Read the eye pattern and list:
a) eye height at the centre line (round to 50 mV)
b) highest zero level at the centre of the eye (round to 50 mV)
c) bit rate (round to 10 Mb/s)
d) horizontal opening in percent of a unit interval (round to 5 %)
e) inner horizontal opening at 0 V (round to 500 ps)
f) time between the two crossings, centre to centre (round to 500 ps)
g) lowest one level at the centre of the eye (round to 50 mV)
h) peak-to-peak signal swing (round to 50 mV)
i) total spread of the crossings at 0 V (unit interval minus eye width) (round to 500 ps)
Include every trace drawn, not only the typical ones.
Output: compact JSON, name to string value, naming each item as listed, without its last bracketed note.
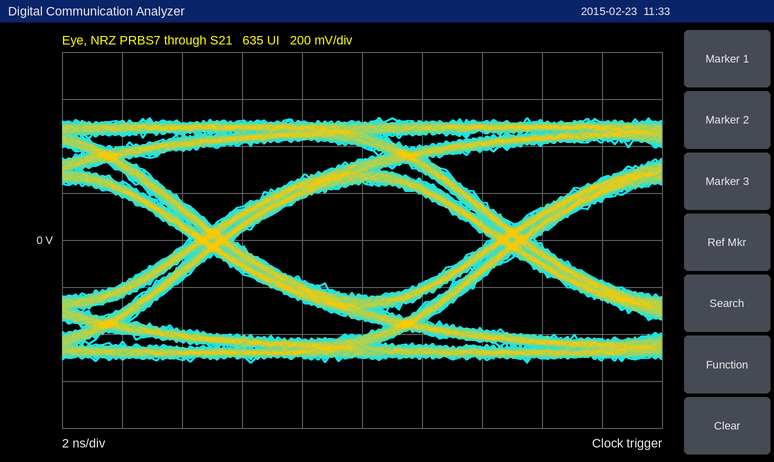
{"eye height at the centre line": "500 mV", "highest zero level at the centre of the eye": "-250 mV", "bit rate": "100 Mb/s", "horizontal opening in percent of a unit interval": "85 %", "inner horizontal opening at 0 V": "8.5 ns", "time between the two crossings, centre to centre": "10.0 ns", "lowest one level at the centre of the eye": "250 mV", "peak-to-peak signal swing": "1.05 V", "total spread of the crossings at 0 V (unit interval minus eye width)": "1.5 ns"}
